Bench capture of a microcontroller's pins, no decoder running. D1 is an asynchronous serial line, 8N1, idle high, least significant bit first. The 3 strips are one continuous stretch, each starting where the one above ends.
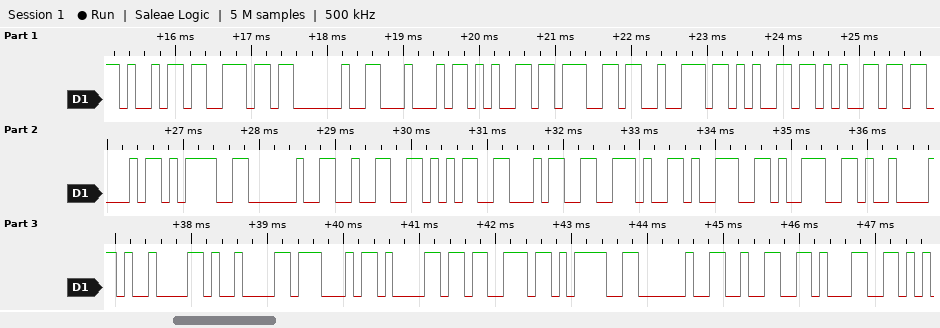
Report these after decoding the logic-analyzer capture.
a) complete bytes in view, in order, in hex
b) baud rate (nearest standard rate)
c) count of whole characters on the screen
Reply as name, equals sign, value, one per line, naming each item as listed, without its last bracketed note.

complete bytes in view, in order, in hex = 0x69 0x6E 0x20 0x44 0x65 0x67 0x72 0x65 0x65 0x43 0x3D 0x20 0x32 0x35 0x34 0x2E 0x39 0x39 0x09 0x09 0x09 0x47 0x61 0x73 0x3D 0x20 0x32 0x31
baud rate = 9600 baud
count of whole characters on the screen = 28
